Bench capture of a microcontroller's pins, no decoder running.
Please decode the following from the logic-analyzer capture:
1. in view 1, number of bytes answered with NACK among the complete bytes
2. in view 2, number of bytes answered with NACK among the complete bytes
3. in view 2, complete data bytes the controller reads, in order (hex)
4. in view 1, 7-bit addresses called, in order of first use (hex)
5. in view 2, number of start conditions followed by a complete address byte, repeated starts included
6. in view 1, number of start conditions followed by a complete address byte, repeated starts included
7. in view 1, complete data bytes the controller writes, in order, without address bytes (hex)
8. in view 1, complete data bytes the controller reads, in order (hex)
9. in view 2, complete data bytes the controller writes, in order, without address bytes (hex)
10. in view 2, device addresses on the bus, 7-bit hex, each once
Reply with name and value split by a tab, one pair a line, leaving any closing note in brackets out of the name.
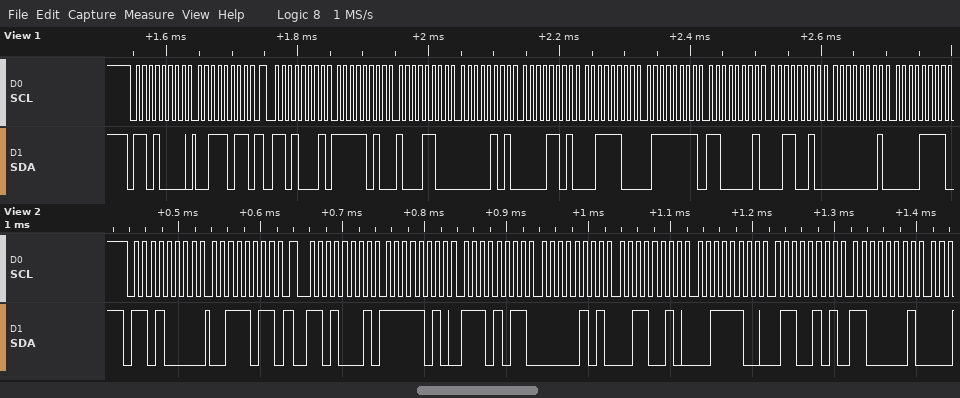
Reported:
in view 1, number of bytes answered with NACK among the complete bytes	0
in view 2, number of bytes answered with NACK among the complete bytes	0
in view 2, complete data bytes the controller reads, in order	FA EB 05 32 3C 65 C1
in view 1, 7-bit addresses called, in order of first use	0x68
in view 2, number of start conditions followed by a complete address byte, repeated starts included	2
in view 1, number of start conditions followed by a complete address byte, repeated starts included	2
in view 1, complete data bytes the controller writes, in order, without address bytes	3B
in view 1, complete data bytes the controller reads, in order	FA 8C 05 0D 3C 7F C1 32 01 0F
in view 2, complete data bytes the controller writes, in order, without address bytes	3B
in view 2, device addresses on the bus, 7-bit hex, each once	0x68
